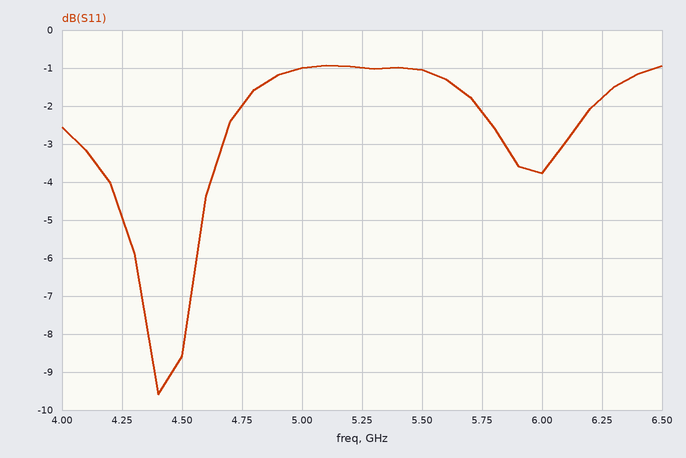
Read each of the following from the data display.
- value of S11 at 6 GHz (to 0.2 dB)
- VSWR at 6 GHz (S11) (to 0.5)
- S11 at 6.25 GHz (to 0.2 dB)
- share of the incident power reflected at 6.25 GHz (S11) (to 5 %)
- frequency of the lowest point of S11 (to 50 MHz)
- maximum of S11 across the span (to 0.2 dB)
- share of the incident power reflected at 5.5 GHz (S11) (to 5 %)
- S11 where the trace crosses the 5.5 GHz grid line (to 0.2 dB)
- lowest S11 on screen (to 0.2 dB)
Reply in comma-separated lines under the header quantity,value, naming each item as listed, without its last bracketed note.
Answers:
quantity,value
value of S11 at 6 GHz,-3.8 dB
VSWR at 6 GHz (S11),4.5
S11 at 6.25 GHz,-1.8 dB
share of the incident power reflected at 6.25 GHz (S11),65 %
frequency of the lowest point of S11,4.40 GHz
maximum of S11 across the span,-1.0 dB
share of the incident power reflected at 5.5 GHz (S11),80 %
S11 where the trace crosses the 5.5 GHz grid line,-1.0 dB
lowest S11 on screen,-9.6 dB
